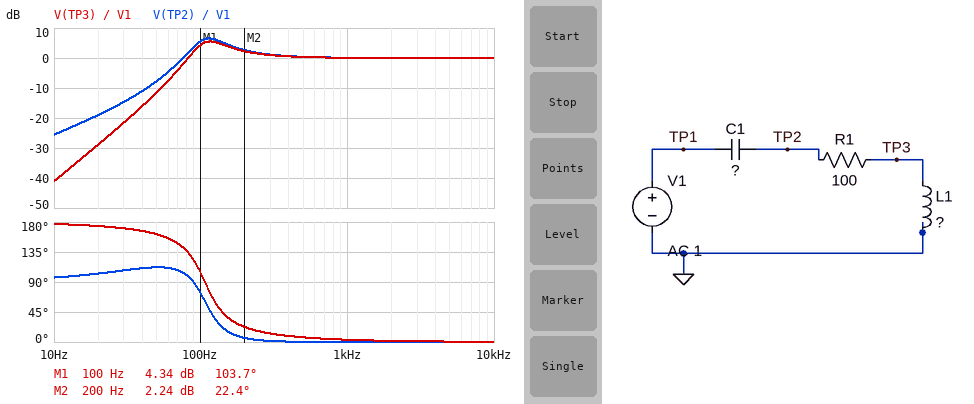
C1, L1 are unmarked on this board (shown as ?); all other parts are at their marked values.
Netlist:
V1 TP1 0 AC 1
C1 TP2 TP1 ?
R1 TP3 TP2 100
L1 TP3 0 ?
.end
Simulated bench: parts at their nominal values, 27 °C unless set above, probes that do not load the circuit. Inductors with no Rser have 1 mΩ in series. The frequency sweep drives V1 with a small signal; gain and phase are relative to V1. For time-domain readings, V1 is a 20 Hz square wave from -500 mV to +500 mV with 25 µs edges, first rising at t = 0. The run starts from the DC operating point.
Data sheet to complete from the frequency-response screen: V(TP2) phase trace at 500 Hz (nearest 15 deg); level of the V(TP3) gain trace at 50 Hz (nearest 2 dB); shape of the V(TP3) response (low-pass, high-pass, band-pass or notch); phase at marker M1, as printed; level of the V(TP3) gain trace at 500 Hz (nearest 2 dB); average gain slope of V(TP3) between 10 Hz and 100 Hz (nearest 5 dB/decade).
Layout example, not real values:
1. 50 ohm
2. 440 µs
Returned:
1. 0 deg
2. -12 dB
3. high-pass
4. 103.7 deg
5. 0 dB
6. 45 dB/decade
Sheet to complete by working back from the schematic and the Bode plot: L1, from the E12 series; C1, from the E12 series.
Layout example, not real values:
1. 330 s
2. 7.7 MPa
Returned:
1. 270 mH
2. 8.2 µF
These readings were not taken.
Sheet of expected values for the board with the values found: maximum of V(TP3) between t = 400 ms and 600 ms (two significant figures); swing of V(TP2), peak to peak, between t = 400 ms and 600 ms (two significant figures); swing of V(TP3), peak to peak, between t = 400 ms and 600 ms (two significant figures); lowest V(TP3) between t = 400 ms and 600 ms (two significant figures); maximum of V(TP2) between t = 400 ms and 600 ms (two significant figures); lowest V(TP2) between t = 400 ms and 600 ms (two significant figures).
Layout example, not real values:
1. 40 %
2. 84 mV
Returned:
1. 1.0 V
2. 2.0 V
3. 2.0 V
4. -1.0 V
5. 1.0 V
6. -1.0 V
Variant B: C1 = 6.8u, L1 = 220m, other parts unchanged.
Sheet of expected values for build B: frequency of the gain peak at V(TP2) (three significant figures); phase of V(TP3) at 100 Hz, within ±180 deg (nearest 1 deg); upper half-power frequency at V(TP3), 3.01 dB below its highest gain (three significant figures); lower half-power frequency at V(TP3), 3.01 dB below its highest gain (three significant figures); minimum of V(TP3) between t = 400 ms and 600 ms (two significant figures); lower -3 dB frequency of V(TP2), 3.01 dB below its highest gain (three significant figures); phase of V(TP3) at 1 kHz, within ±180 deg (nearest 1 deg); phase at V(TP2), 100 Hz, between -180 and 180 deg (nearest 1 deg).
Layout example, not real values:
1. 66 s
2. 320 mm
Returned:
1. 139 Hz
2. 134 deg
3. 233 Hz
4. 111 Hz
5. -990 mV
6. 108 Hz
7. 4 deg
8. 98 deg
